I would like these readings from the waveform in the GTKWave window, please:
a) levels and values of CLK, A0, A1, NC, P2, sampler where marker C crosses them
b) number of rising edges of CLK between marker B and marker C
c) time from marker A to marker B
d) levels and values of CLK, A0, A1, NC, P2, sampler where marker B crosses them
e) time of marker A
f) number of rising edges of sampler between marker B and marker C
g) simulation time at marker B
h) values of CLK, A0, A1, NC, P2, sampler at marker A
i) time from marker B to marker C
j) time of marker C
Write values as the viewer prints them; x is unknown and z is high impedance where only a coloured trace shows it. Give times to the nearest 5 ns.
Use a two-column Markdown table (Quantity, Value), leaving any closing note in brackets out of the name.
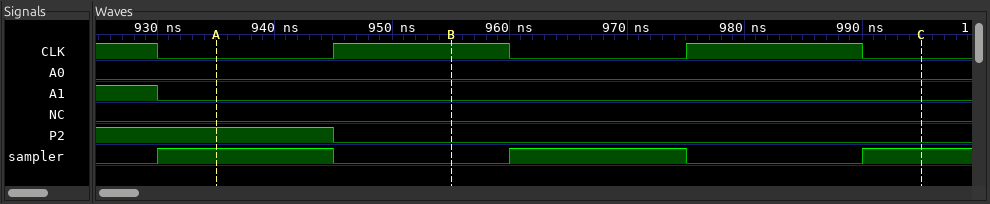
| Quantity | Value |
|---|---|
| levels and values of CLK, A0, A1, NC, P2, sampler where marker C crosses them | CLK=0, A0=0, A1=0, NC=0, P2=0, sampler=1 |
| number of rising edges of CLK between marker B and marker C | 1 |
| time from marker A to marker B | 20 ns |
| levels and values of CLK, A0, A1, NC, P2, sampler where marker B crosses them | CLK=1, A0=0, A1=0, NC=0, P2=0, sampler=0 |
| time of marker A | 935 ns |
| number of rising edges of sampler between marker B and marker C | 2 |
| simulation time at marker B | 955 ns |
| values of CLK, A0, A1, NC, P2, sampler at marker A | CLK=0, A0=0, A1=0, NC=0, P2=1, sampler=1 |
| time from marker B to marker C | 40 ns |
| time of marker C | 995 ns |
